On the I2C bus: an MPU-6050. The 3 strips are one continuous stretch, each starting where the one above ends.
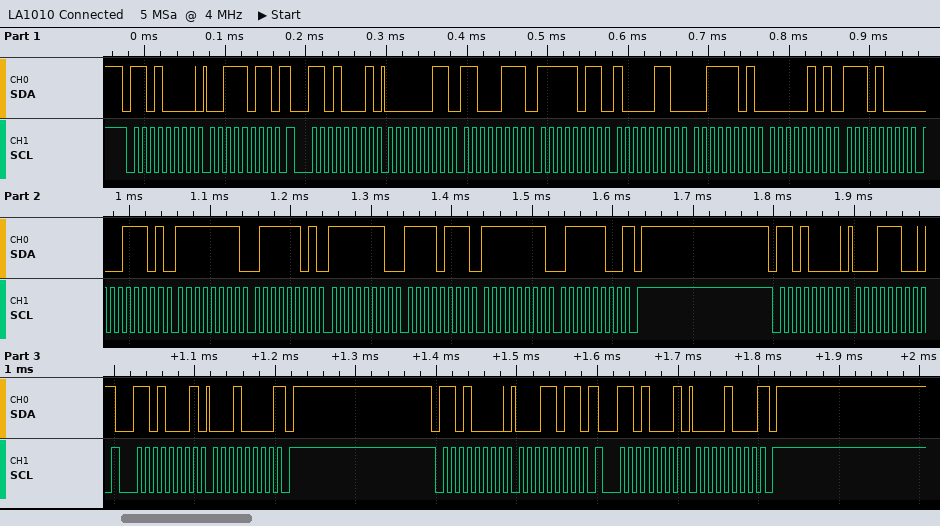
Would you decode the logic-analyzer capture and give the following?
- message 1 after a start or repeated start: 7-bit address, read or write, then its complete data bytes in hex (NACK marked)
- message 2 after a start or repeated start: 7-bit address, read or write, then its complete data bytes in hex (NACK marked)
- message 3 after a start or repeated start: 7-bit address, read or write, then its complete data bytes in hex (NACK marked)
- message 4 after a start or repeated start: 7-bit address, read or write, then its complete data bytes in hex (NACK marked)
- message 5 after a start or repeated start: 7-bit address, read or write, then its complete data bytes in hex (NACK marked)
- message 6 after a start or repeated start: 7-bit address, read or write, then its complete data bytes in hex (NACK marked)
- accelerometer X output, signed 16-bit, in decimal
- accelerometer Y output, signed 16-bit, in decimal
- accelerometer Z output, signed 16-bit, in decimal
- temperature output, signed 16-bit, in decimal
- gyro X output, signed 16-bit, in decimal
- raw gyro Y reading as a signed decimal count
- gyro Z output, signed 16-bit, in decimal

0x68 write: 3B
0x68 read: 03 C7 FB 86 3D 05 E8 1D FF 7D FE F7 FF 7C NACK
0x68 write: 1C
0x68 read: 10 NACK
0x68 write: 1B
0x68 read: 08 NACK
967
-1146
15621
-6115
-131
-265
-132
